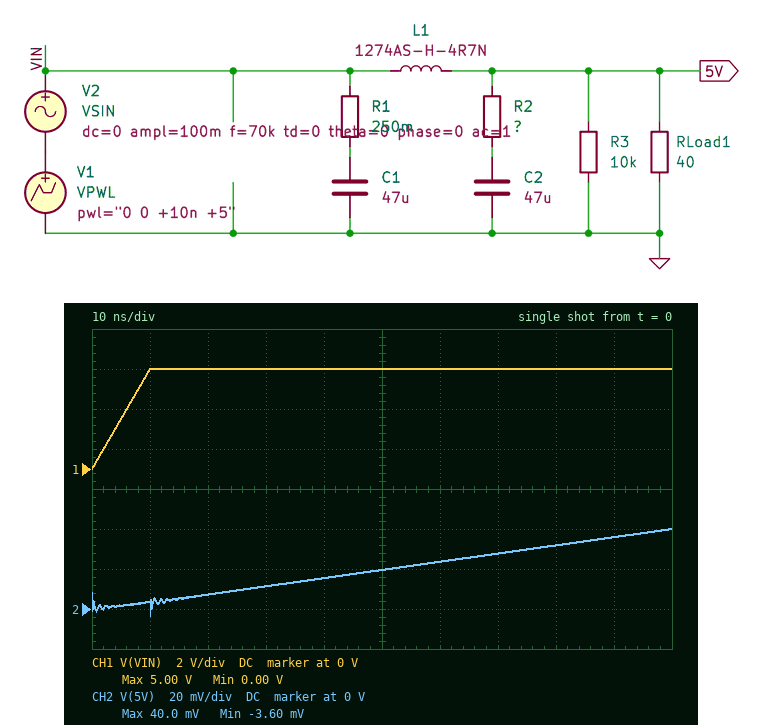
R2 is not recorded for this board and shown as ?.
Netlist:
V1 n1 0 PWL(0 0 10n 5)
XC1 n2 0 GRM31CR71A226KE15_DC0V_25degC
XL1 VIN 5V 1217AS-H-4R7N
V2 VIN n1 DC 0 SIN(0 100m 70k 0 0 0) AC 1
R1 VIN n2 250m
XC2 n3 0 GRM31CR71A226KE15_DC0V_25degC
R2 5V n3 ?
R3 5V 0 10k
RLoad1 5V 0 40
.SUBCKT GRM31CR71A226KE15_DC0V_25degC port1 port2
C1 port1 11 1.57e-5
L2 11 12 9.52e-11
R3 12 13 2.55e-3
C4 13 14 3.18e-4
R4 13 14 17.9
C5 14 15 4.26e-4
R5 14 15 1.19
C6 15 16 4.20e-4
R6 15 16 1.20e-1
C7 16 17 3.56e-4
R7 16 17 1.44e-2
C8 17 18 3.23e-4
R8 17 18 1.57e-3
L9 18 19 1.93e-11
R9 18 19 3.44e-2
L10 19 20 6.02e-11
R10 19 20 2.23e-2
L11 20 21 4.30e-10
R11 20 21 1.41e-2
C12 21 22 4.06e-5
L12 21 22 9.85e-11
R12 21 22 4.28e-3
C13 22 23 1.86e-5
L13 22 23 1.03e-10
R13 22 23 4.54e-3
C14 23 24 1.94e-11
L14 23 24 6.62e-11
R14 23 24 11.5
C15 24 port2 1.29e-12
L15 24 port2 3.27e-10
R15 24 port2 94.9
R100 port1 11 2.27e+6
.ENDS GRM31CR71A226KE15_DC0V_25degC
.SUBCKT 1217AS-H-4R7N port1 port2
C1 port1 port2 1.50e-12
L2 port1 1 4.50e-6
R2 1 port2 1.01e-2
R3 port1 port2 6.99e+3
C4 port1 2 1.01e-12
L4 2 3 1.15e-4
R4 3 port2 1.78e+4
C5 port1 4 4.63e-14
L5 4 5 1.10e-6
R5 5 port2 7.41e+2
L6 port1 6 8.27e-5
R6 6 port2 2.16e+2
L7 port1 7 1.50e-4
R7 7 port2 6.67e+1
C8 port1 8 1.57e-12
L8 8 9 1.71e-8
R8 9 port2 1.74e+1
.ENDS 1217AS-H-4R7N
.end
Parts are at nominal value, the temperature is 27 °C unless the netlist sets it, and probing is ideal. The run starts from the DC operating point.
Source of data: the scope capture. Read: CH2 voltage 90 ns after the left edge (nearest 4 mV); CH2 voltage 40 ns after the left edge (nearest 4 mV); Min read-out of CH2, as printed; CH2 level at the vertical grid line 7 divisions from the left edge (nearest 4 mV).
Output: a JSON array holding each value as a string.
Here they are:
["36 mV", "16 mV", "-3.60 mV", "28 mV"]
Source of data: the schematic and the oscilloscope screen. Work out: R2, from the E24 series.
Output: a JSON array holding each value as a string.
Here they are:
["0.33 Ω"]
